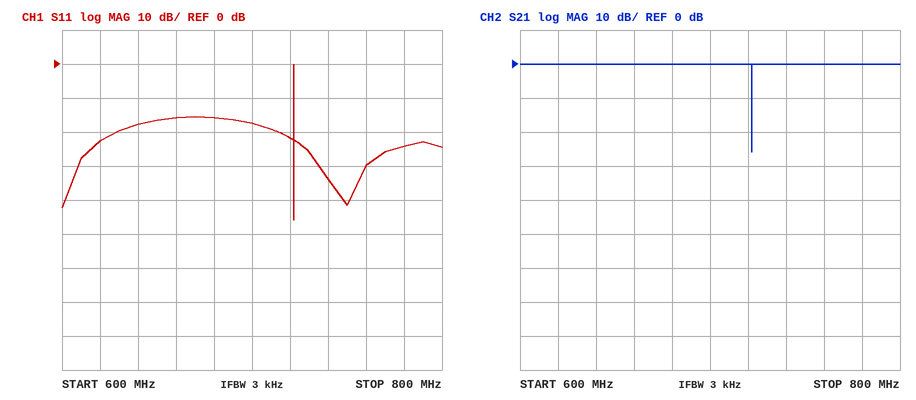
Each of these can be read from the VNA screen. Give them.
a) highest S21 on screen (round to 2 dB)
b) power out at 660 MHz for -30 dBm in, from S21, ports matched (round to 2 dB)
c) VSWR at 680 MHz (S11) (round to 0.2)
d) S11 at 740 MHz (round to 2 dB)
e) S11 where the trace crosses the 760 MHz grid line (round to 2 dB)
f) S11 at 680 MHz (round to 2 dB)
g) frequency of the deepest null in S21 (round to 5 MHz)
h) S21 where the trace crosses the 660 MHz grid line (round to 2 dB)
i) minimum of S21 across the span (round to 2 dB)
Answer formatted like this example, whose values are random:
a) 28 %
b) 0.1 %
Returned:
a) 0 dB
b) -30 dBm
c) 1.4
d) -34 dB
e) -30 dB
f) -16 dB
g) 720 MHz
h) 0 dB
i) -26 dB
